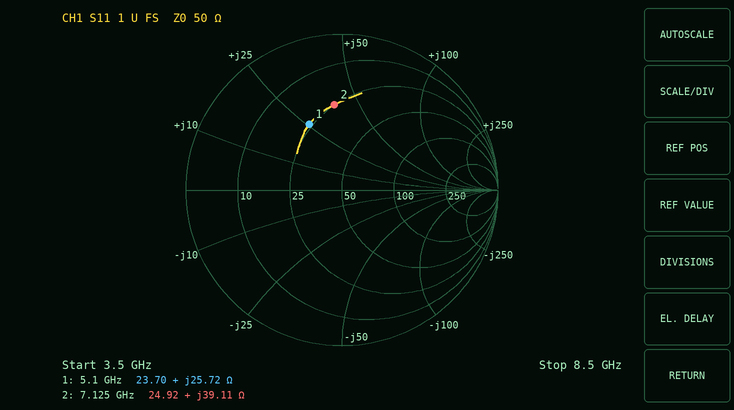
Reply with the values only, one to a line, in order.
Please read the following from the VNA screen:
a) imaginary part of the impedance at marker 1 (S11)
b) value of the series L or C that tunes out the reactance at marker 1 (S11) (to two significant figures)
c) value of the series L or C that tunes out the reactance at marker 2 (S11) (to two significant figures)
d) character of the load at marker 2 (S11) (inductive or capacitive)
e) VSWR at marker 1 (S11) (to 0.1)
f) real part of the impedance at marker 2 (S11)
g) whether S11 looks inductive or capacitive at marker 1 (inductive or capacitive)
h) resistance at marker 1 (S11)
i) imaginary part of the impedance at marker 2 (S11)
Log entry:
+25.72 Ω
1.2 pF
570 fF
inductive
2.8
24.92 Ω
inductive
23.70 Ω
+39.11 Ω
